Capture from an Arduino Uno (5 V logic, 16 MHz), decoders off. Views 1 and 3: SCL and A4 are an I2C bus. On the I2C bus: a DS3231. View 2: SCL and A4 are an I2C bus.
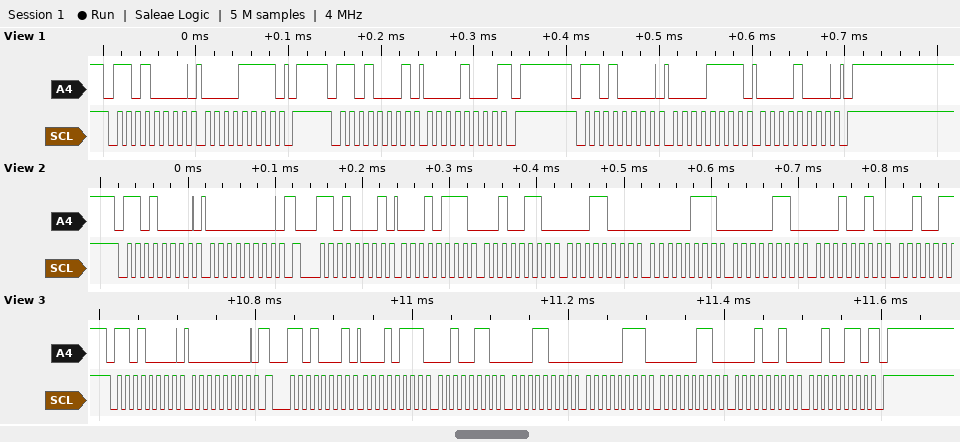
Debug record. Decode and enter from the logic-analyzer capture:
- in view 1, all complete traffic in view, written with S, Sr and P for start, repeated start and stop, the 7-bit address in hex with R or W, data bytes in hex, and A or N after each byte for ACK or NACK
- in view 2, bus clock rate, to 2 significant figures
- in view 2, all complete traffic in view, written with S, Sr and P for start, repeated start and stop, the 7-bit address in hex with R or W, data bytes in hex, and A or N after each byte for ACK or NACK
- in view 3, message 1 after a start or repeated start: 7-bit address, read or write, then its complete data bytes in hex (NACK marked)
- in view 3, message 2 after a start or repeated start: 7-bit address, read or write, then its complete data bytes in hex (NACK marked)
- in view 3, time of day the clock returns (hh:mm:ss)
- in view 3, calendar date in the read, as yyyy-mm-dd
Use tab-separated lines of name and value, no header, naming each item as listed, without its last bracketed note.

in view 1, all complete traffic in view, written with S, Sr and P for start, repeated start and stop, the 7-bit address in hex with R or W, data bytes in hex, and A or N after each byte for ACK or NACK	S 68W A 0F A P S 68R A 08 N P S 68W A 0F A 08 A P
in view 2, bus clock rate, to 2 significant figures	100 kHz
in view 2, all complete traffic in view, written with S, Sr and P for start, repeated start and stop, the 7-bit address in hex with R or W, data bytes in hex, and A or N after each byte for ACK or NACK	S 68W A 00 A Sr 68R A 17 A 26 A 18 A 07 A 06 A 12 A
in view 3, message 1 after a start or repeated start: 7-bit address, read or write, then its complete data bytes in hex	0x68 write: 00
in view 3, message 2 after a start or repeated start: 7-bit address, read or write, then its complete data bytes in hex	0x68 read: 17 26 18 07 06 12 26 NACK
in view 3, time of day the clock returns	18:26:17
in view 3, calendar date in the read, as yyyy-mm-dd	2026-12-06
